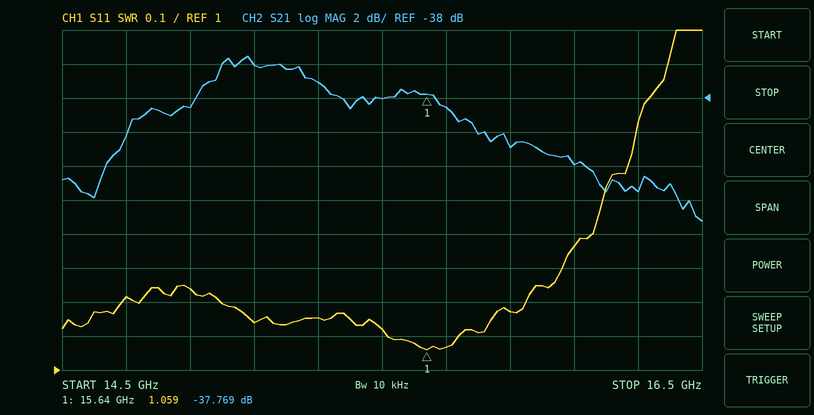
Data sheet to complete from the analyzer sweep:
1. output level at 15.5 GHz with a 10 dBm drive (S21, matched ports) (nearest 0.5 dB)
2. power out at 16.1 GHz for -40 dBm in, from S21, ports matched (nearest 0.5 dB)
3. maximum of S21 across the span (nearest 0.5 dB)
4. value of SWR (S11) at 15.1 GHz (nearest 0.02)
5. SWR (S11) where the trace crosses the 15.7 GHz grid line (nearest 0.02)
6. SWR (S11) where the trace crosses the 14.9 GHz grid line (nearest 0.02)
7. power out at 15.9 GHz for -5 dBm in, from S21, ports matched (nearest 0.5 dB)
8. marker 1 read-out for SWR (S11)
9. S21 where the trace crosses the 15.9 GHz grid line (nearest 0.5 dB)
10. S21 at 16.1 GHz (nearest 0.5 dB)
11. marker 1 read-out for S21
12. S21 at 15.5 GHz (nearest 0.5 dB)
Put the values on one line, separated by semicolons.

-28.0 dBm; -82.0 dBm; -35.5 dB; 1.14; 1.06; 1.24; -46.0 dBm; 1.059; -41.0 dB; -42.0 dB; -37.769 dB; -38.0 dB
